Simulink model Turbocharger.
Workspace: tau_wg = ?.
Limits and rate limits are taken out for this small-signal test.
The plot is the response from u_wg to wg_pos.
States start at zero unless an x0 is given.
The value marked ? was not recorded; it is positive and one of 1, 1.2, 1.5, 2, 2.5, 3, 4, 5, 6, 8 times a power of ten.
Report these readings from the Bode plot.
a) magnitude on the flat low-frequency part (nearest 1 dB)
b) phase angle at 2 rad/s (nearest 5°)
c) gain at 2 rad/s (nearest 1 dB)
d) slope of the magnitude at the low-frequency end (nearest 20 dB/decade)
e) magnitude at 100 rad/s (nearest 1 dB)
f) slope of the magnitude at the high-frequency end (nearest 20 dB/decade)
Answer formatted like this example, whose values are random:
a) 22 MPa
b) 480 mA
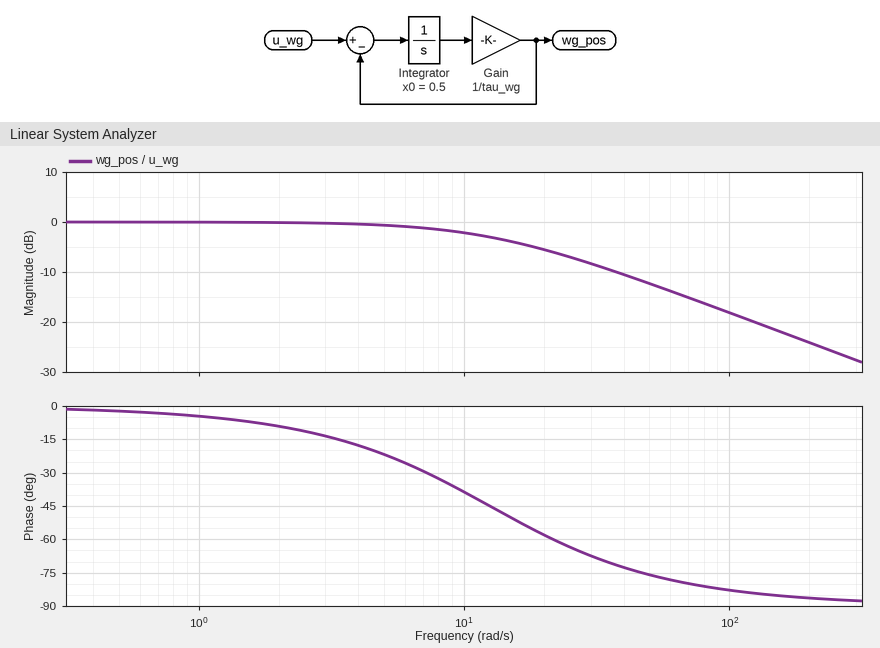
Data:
a) 0 dB
b) -10°
c) 0 dB
d) 0 dB/decade
e) -18 dB
f) -20 dB/decade
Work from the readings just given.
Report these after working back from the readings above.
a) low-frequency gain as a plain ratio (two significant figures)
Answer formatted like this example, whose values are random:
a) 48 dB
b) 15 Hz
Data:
a) 1.0
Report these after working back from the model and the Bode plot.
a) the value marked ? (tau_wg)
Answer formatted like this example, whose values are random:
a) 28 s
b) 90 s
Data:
a) 0.08
